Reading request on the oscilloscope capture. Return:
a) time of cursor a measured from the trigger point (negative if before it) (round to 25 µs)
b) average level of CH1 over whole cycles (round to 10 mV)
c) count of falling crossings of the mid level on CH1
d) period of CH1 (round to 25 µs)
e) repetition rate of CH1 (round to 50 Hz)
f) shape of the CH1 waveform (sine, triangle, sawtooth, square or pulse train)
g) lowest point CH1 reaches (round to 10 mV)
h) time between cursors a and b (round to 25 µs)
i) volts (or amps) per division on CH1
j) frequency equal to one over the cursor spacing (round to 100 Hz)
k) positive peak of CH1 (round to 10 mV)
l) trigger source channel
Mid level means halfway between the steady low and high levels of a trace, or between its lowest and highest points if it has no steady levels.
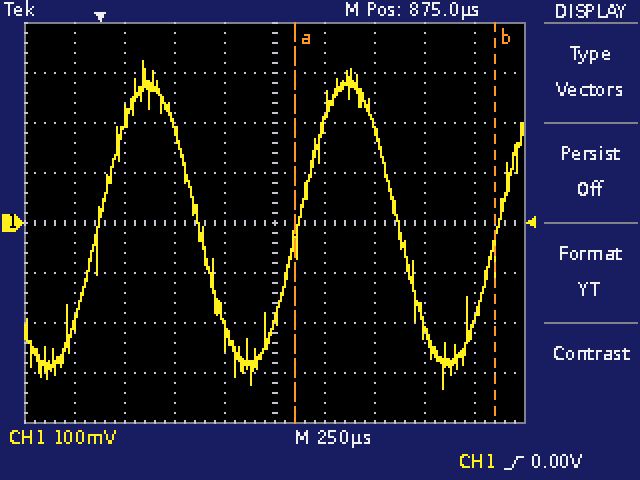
+975 µs
0 mV
2
1.000 ms
1.00 kHz
sine
-330 mV
1.000 ms
100 mV
1.0 kHz
320 mV
CH1
